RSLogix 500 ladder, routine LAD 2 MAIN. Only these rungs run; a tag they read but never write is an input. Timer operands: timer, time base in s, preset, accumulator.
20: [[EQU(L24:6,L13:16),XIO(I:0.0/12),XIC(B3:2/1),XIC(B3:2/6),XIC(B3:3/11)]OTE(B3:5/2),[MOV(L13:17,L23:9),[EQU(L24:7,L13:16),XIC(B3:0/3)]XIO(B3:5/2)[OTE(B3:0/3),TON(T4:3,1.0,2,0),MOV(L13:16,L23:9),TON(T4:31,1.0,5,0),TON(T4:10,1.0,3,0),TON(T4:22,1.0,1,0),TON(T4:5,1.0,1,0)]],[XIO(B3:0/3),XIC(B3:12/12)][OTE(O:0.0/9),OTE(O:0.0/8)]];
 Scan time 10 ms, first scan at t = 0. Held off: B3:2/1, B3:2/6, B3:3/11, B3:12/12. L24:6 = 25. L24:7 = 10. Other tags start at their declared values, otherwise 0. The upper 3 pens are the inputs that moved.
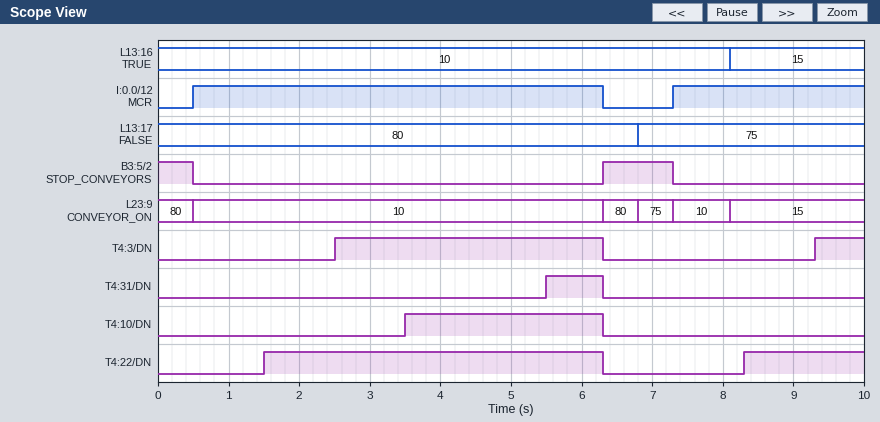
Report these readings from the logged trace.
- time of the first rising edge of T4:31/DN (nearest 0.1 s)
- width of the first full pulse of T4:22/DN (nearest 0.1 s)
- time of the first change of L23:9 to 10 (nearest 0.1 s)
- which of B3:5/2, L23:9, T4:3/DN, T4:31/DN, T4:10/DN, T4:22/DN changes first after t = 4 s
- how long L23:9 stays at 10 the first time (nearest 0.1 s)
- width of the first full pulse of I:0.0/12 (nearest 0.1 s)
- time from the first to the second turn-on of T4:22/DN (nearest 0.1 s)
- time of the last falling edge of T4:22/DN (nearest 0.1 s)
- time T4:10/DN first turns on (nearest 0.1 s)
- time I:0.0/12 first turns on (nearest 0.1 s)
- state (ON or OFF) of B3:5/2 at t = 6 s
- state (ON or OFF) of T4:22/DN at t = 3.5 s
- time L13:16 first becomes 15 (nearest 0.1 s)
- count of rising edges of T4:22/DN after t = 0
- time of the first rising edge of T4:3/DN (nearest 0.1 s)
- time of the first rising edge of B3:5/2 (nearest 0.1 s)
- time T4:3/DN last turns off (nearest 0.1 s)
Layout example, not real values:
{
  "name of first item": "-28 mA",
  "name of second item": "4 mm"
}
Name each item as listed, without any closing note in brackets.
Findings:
{
  "time of the first rising edge of T4:31/DN": "5.5 s",
  "width of the first full pulse of T4:22/DN": "4.8 s",
  "time of the first change of L23:9 to 10": "0.5 s",
  "which of B3:5/2, L23:9, T4:3/DN, T4:31/DN, T4:10/DN, T4:22/DN changes first after t = 4 s": "T4:31/DN",
  "how long L23:9 stays at 10 the first time": "5.8 s",
  "width of the first full pulse of I:0.0/12": "5.8 s",
  "time from the first to the second turn-on of T4:22/DN": "6.8 s",
  "time of the last falling edge of T4:22/DN": "6.3 s",
  "time T4:10/DN first turns on": "3.5 s",
  "time I:0.0/12 first turns on": "0.5 s",
  "state (ON or OFF) of B3:5/2 at t = 6 s": "OFF",
  "state (ON or OFF) of T4:22/DN at t = 3.5 s": "ON",
  "time L13:16 first becomes 15": "8.1 s",
  "count of rising edges of T4:22/DN after t = 0": "2",
  "time of the first rising edge of T4:3/DN": "2.5 s",
  "time of the first rising edge of B3:5/2": "6.3 s",
  "time T4:3/DN last turns off": "6.3 s"
}
